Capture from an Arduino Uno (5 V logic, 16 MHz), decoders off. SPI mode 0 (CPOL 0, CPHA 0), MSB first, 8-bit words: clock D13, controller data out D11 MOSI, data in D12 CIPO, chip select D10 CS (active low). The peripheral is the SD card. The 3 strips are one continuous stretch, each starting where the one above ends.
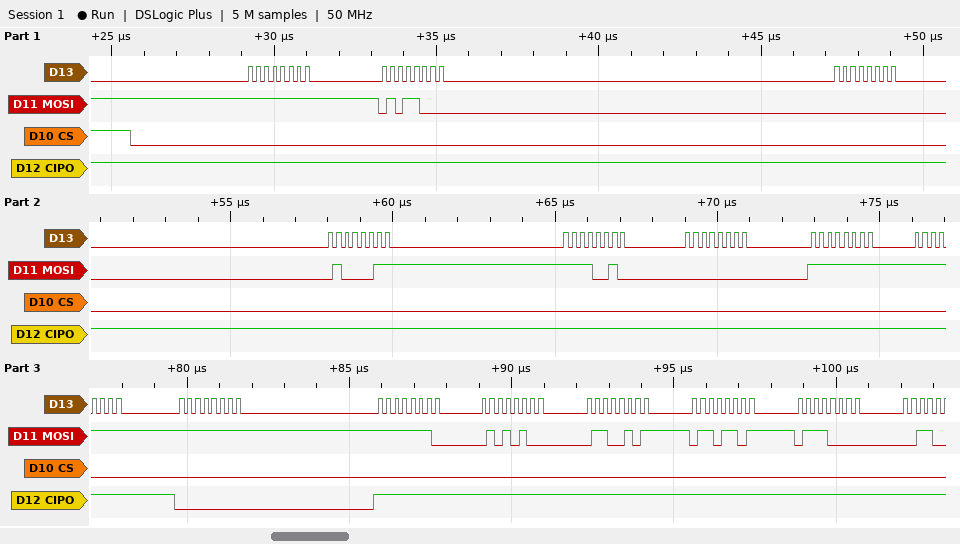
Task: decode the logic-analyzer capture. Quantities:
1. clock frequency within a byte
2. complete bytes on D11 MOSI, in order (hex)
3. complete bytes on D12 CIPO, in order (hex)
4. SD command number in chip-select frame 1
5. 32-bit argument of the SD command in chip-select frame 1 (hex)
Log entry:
4 MHz
0xFF 0x58 0x00 0x43 0xF2 0x00 0xFF 0xFF 0xFF 0xFE 0x54 0x65 0x6D 0x70
0xFF 0xFF 0xFF 0xFF 0xFF 0xFF 0xFF 0xFF 0x00 0xFF 0xFF 0xFF 0xFF 0xFF
CMD24
0x0043F200
